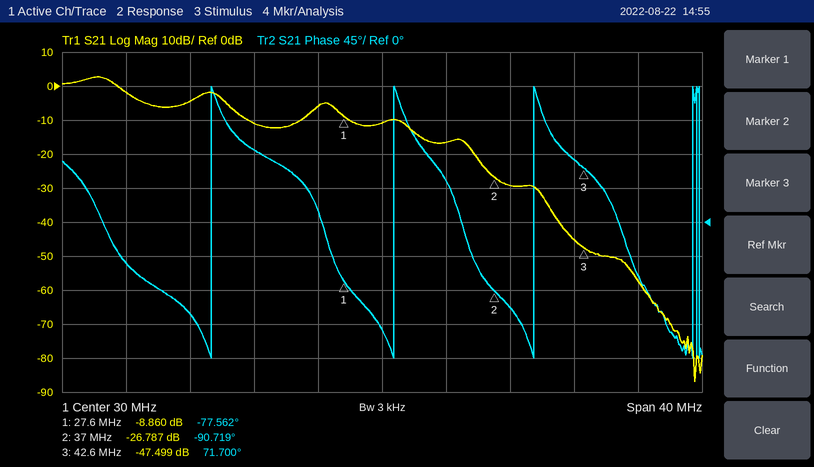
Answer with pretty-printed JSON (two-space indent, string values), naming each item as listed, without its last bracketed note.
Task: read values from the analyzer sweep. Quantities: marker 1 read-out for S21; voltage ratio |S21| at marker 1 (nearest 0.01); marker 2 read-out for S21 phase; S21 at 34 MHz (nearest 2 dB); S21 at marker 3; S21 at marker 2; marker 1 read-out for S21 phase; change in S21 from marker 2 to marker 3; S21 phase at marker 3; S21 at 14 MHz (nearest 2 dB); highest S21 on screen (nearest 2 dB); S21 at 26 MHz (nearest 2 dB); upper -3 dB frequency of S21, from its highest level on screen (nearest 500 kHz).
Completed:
{
  "marker 1 read-out for S21": "-8.860 dB",
  "voltage ratio |S21| at marker 1": "0.36",
  "marker 2 read-out for S21 phase": "-90.719°",
  "S21 at 34 MHz": "-16 dB",
  "S21 at marker 3": "-47.499 dB",
  "S21 at marker 2": "-26.787 dB",
  "marker 1 read-out for S21 phase": "-77.562°",
  "change in S21 from marker 2 to marker 3": "-20.712 dB",
  "S21 phase at marker 3": "71.700°",
  "S21 at 14 MHz": "-2 dB",
  "highest S21 on screen": "2 dB",
  "S21 at 26 MHz": "-6 dB",
  "upper -3 dB frequency of S21, from its highest level on screen": "13.5 MHz"
}
